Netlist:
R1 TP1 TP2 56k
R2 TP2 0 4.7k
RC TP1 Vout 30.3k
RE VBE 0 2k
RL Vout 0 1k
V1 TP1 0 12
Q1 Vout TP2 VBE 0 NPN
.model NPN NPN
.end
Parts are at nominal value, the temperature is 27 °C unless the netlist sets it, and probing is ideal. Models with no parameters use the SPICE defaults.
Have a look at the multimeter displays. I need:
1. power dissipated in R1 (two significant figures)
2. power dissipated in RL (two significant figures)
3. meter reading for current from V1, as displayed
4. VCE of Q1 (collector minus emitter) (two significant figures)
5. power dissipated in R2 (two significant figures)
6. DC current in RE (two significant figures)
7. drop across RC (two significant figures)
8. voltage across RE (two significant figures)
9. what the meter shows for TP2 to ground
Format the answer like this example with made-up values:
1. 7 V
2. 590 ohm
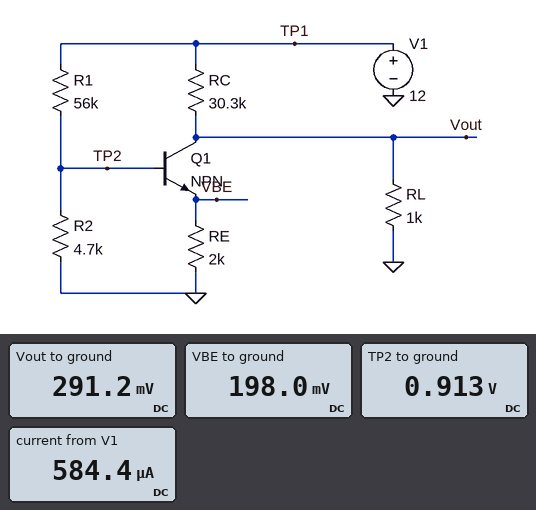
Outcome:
1. 2.2 mW
2. 85 µW
3. 584.4 µA
4. 93 mV
5. 180 µW
6. 99 µA
7. 12 V
8. 200 mV
9. 0.913 V
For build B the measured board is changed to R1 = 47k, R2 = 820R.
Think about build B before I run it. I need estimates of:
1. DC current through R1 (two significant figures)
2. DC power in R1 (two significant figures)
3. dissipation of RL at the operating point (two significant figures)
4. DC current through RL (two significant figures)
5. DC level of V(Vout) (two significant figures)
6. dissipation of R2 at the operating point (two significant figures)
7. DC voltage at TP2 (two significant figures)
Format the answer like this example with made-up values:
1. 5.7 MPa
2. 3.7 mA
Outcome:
1. 250 µA
2. 3.0 mW
3. 150 µW
4. 380 µA
5. 380 mV
6. 52 µW
7. 210 mV
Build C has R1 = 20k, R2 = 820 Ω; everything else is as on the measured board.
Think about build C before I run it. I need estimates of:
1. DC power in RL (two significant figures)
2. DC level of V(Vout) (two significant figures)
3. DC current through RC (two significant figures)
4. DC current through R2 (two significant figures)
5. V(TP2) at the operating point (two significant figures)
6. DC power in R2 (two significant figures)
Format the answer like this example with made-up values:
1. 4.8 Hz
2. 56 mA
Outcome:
1. 150 µW
2. 380 mV
3. 380 µA
4. 580 µA
5. 470 mV
6. 270 µW
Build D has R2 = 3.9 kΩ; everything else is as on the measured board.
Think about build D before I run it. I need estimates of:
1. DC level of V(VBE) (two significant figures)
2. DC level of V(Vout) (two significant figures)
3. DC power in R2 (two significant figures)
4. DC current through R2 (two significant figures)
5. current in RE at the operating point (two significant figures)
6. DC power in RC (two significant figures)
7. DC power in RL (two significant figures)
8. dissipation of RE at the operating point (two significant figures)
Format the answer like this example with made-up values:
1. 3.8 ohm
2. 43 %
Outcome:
1. 87 mV
2. 340 mV
3. 160 µW
4. 200 µA
5. 43 µA
6. 4.5 mW
7. 120 µW
8. 3.8 µW
